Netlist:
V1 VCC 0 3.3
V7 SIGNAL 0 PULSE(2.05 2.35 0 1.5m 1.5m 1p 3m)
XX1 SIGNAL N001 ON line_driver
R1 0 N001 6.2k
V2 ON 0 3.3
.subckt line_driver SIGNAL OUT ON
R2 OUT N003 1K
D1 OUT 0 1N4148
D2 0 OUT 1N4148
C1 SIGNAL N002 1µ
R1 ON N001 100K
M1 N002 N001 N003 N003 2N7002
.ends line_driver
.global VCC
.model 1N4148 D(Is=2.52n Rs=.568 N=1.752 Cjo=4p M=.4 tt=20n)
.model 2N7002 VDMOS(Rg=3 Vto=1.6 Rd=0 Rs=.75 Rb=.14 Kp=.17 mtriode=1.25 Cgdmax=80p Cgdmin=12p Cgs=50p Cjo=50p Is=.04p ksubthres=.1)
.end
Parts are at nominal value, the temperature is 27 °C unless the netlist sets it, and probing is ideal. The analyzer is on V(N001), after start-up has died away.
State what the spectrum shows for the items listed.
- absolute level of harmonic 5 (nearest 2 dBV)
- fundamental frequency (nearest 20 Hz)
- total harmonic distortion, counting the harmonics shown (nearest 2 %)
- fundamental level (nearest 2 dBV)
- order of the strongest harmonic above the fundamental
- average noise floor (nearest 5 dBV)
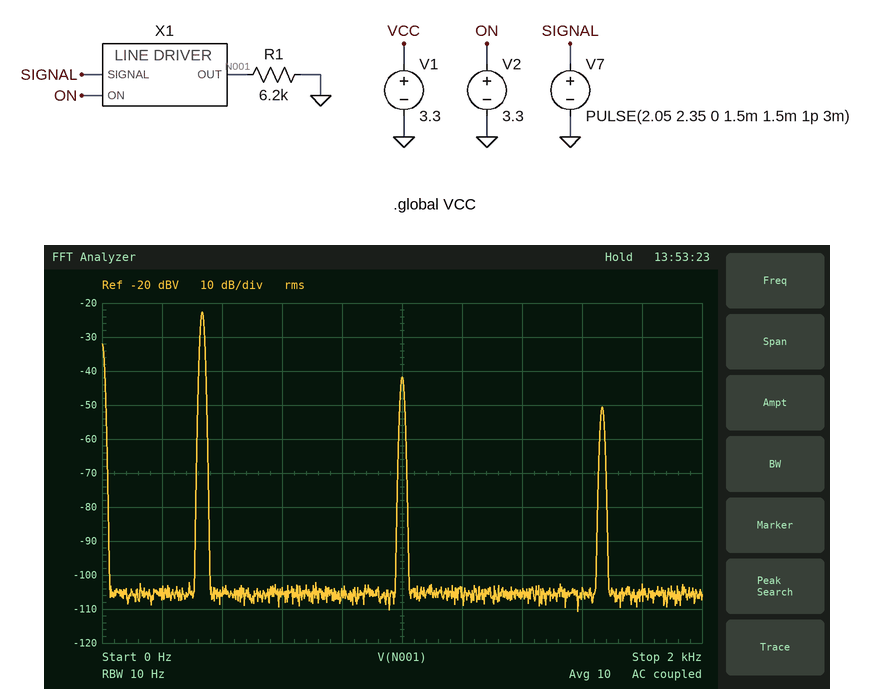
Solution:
-50 dBV
340 Hz
12 %
-22 dBV
3
-105 dBV
